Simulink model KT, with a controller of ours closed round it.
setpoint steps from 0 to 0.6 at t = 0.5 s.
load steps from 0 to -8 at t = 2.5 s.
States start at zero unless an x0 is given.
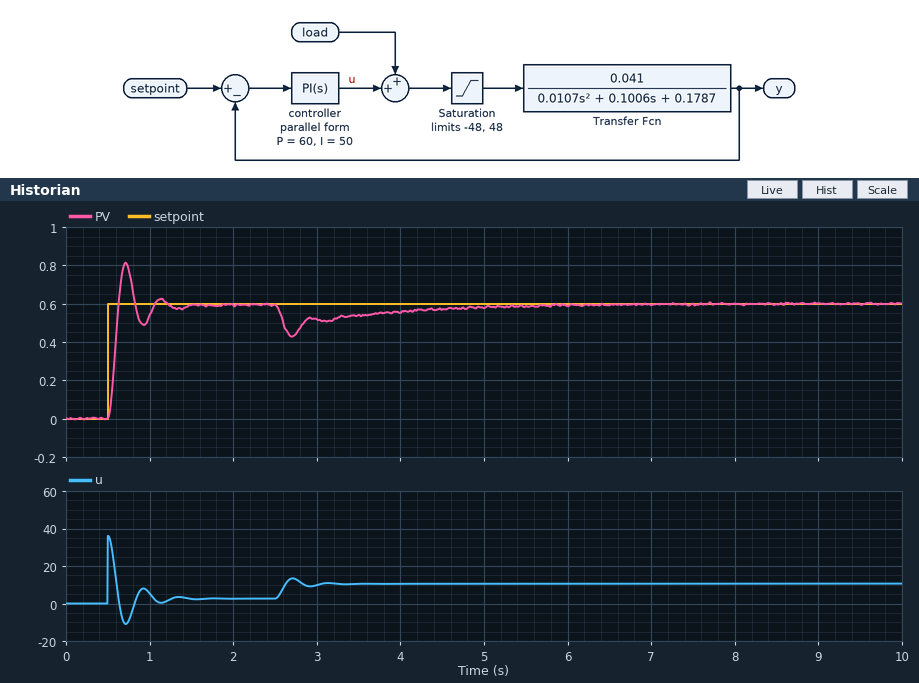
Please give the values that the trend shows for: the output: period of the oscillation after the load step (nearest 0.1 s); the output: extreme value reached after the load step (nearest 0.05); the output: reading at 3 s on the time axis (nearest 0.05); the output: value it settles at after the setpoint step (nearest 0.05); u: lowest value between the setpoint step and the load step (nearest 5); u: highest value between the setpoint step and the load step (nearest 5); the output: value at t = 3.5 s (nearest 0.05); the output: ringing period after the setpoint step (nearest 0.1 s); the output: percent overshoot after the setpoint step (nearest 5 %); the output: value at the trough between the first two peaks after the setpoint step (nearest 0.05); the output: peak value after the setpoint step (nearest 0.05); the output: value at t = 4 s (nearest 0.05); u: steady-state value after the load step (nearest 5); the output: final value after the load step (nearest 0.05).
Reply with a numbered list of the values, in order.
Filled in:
1. 0.4 s
2. 0.45
3. 0.50
4. 0.60
5. -10
6. 35
7. 0.55
8. 0.4 s
9. 35 %
10. 0.50
11. 0.80
12. 0.55
13. 10
14. 0.60
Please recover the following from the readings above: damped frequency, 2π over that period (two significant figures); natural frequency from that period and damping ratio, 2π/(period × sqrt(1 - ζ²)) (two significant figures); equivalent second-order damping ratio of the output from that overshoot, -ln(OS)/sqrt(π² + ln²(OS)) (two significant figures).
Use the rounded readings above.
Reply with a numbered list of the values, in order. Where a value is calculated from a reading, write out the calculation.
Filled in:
1. 2π / 0.4 = 16 rad/s
2. 2π / (0.4 × sqrt(1 - 0.32²)) = 17 rad/s
3. ln(0.35) = -1.050; 1.050 / sqrt(9.870 + 1.102) = 0.32
